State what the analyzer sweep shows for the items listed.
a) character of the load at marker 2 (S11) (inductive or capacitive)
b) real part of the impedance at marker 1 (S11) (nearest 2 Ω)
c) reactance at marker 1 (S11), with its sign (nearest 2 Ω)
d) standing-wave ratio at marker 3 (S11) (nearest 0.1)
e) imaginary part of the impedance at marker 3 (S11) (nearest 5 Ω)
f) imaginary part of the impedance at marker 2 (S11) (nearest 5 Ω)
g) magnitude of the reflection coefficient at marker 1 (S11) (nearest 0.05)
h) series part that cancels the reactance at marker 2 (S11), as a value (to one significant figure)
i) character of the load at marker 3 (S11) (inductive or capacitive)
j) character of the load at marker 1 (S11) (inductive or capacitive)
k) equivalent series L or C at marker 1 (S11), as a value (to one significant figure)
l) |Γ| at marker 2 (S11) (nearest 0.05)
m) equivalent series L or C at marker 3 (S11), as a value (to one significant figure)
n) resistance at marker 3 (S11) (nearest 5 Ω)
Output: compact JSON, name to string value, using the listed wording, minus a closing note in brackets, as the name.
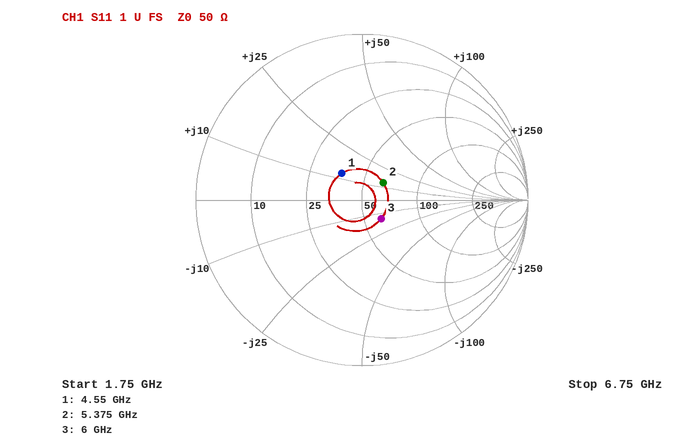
{"character of the load at marker 2 (S11)": "inductive", "real part of the impedance at marker 1 (S11)": "38 Ω", "reactance at marker 1 (S11), with its sign": "+12 Ω", "standing-wave ratio at marker 3 (S11)": "1.4", "imaginary part of the impedance at marker 3 (S11)": "-15 Ω", "imaginary part of the impedance at marker 2 (S11)": "+15 Ω", "magnitude of the reflection coefficient at marker 1 (S11)": "0.20", "series part that cancels the reactance at marker 2 (S11), as a value": "2 pF", "character of the load at marker 3 (S11)": "capacitive", "character of the load at marker 1 (S11)": "inductive", "equivalent series L or C at marker 1 (S11), as a value": "400 pH", "|Γ| at marker 2 (S11)": "0.15", "equivalent series L or C at marker 3 (S11), as a value": "2 pF", "resistance at marker 3 (S11)": "60 Ω"}
